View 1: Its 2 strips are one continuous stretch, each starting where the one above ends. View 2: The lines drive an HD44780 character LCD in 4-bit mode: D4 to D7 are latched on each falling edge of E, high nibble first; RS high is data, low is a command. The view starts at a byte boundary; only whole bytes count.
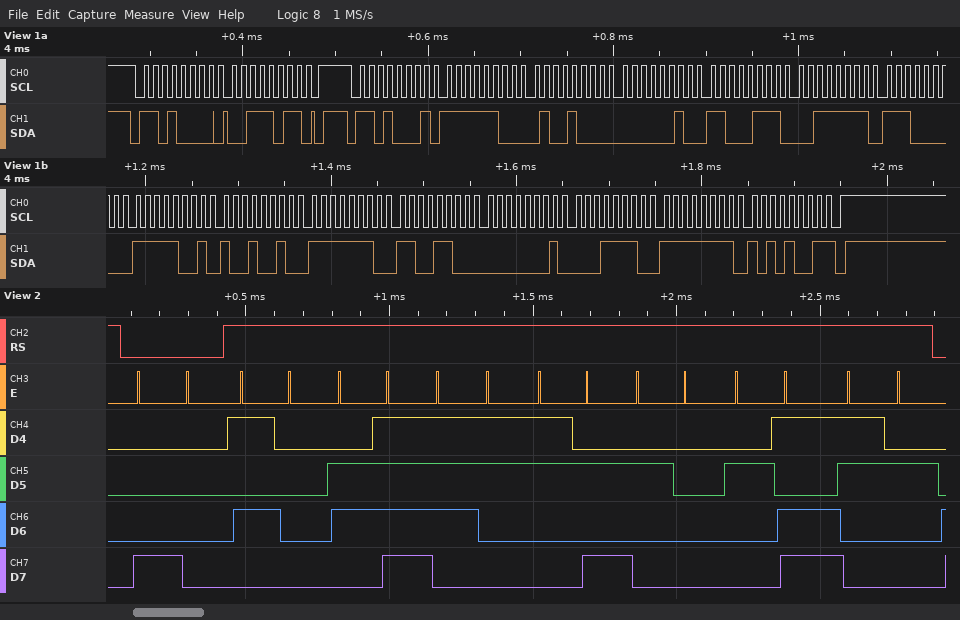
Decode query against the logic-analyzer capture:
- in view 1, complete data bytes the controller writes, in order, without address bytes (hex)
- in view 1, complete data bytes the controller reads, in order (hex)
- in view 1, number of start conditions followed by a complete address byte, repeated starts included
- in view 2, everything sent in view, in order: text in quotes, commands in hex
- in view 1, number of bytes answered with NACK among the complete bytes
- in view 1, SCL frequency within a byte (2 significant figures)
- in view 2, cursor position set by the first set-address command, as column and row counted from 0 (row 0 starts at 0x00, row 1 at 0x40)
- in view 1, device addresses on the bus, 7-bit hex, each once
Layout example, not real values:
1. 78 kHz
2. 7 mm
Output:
1. 3B
2. FC 48 02 C7 3F E0 F9 92 FE CC 01 1E FF A9
3. 2
4. 0x80 "Pos: -2"
5. 1
6. 100 kHz
7. column 0, row 0
8. 0x68
